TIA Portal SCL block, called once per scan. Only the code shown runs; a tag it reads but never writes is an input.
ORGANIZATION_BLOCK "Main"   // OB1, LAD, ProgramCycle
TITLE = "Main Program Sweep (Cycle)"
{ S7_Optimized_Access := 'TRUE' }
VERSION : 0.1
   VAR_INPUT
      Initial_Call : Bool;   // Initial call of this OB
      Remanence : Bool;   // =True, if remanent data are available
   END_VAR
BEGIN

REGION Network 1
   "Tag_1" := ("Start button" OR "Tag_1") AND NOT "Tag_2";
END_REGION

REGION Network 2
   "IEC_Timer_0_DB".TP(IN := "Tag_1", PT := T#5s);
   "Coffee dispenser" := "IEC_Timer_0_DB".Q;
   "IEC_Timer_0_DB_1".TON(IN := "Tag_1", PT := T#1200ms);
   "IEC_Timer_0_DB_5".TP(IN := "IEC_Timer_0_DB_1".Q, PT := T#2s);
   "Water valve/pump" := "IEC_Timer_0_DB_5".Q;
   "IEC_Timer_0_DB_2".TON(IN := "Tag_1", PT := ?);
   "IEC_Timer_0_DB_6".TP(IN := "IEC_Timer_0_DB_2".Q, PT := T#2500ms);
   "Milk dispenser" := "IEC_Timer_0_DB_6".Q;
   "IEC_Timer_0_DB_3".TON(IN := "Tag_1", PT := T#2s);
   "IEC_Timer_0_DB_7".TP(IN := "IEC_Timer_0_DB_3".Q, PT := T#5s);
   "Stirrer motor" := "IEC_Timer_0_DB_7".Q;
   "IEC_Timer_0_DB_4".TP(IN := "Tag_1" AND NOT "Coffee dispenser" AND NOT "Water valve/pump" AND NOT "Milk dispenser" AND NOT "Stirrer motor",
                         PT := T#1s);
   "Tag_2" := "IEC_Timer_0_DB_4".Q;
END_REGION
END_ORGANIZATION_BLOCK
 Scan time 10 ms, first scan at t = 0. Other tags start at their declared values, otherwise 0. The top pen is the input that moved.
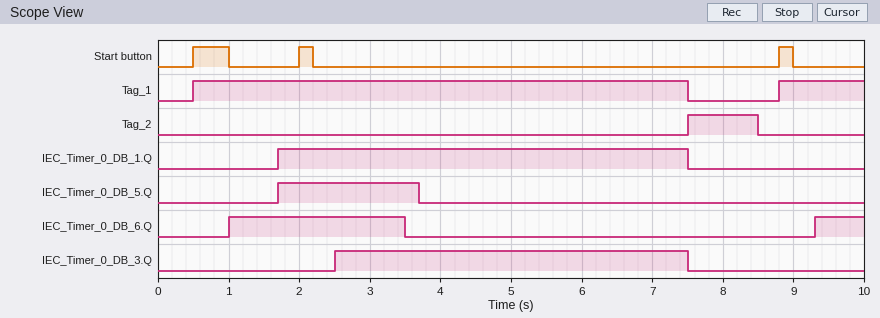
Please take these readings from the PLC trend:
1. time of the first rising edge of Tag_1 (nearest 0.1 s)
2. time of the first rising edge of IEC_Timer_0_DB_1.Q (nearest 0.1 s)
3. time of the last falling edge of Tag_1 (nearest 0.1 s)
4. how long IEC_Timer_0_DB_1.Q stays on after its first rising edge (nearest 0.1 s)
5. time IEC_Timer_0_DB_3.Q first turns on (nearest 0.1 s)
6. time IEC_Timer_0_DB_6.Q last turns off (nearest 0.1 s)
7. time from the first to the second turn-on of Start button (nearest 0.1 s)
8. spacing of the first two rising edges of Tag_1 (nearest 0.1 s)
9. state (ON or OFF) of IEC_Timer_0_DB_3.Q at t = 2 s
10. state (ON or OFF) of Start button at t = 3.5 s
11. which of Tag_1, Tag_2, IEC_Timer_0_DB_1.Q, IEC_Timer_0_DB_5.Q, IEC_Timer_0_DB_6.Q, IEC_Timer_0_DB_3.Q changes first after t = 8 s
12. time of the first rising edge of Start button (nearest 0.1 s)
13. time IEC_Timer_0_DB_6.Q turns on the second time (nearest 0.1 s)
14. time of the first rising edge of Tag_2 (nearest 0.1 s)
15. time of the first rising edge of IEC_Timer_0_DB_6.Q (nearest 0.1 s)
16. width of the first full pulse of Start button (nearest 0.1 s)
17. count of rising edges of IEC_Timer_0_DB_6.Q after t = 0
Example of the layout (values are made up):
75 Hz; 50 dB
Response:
0.5 s; 1.7 s; 7.5 s; 5.8 s; 2.5 s; 3.5 s; 1.5 s; 8.3 s; OFF; OFF; Tag_2; 0.5 s; 9.3 s; 7.5 s; 1.0 s; 0.5 s; 2
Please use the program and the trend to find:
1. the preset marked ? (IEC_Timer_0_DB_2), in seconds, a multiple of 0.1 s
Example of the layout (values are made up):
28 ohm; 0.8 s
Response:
0.5 s
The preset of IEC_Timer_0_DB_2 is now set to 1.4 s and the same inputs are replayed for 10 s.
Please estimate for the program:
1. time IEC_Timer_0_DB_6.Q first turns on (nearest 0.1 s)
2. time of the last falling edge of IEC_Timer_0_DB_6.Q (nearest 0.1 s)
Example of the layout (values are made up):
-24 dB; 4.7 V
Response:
1.9 s; 4.4 s
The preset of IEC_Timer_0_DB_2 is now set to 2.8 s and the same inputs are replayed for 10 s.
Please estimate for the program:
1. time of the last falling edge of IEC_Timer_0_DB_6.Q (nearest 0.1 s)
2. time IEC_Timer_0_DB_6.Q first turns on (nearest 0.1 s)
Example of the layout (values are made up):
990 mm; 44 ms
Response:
5.8 s; 3.3 s
